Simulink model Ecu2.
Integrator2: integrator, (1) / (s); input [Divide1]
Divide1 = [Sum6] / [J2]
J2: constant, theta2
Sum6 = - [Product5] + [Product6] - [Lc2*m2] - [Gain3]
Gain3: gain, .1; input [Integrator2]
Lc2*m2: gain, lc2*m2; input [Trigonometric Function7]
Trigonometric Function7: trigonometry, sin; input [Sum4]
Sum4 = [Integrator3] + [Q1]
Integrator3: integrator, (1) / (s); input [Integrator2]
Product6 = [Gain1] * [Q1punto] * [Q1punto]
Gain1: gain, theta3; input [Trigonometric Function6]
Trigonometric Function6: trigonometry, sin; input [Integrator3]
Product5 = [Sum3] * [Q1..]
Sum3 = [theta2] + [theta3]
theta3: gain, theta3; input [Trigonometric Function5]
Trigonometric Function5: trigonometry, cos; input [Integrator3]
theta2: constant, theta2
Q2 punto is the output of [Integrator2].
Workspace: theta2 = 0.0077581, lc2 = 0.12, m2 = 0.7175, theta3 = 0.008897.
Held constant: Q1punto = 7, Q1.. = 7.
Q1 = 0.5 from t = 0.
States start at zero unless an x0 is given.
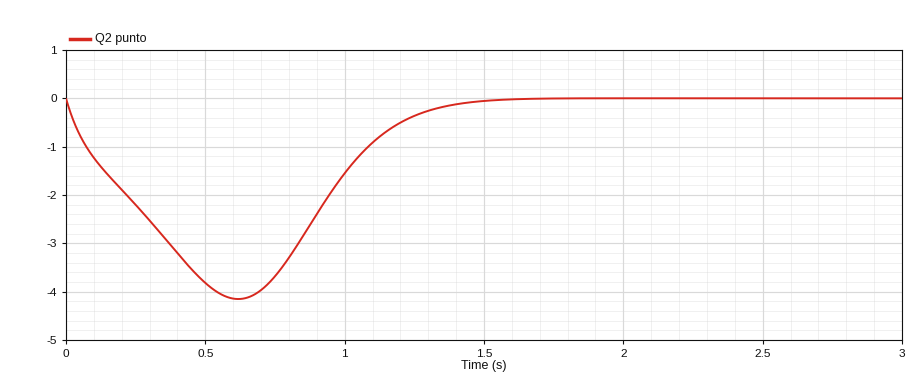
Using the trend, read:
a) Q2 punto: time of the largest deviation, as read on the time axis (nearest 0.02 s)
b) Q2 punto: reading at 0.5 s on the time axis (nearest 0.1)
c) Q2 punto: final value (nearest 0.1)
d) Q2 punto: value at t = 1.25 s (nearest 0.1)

0.62 s
-3.8
0.0
-0.4
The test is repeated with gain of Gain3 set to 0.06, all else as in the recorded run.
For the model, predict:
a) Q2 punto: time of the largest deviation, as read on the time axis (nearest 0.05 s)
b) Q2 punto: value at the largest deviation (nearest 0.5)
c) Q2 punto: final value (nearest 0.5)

0.50 s
-6.5
0.0
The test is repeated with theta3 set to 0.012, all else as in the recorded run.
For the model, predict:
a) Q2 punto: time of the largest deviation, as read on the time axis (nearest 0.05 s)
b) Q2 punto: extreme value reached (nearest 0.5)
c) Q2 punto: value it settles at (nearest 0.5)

0.55 s
-5.5
0.0
